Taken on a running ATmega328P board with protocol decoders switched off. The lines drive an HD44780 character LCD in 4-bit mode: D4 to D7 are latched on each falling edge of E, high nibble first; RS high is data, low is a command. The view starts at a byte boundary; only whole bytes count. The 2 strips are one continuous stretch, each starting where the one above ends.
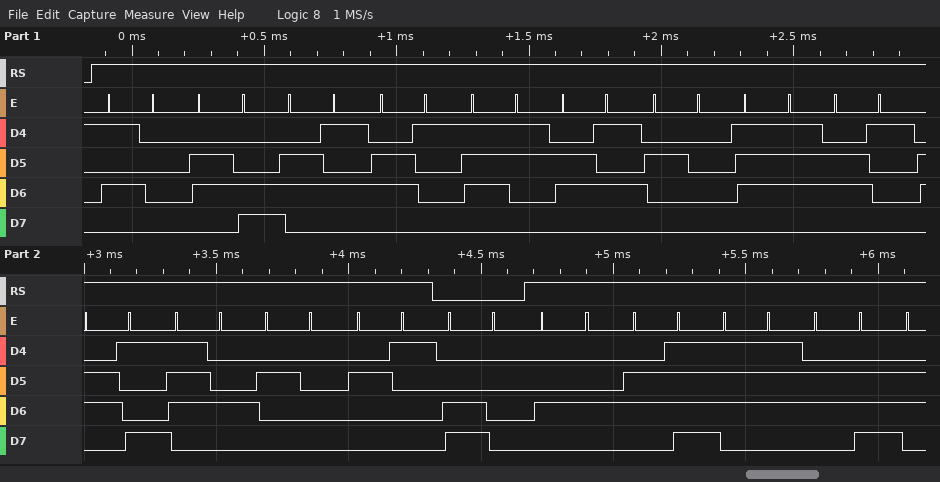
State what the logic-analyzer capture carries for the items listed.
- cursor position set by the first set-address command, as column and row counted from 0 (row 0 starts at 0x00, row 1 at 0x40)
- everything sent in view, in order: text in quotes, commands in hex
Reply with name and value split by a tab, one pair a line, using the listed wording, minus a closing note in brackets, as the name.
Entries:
cursor position set by the first set-address command, as column and row counted from 0	column 0, row 1
everything sent in view, in order: text in quotes, commands in hex	"Please wait !" 0xC0 "Down"
